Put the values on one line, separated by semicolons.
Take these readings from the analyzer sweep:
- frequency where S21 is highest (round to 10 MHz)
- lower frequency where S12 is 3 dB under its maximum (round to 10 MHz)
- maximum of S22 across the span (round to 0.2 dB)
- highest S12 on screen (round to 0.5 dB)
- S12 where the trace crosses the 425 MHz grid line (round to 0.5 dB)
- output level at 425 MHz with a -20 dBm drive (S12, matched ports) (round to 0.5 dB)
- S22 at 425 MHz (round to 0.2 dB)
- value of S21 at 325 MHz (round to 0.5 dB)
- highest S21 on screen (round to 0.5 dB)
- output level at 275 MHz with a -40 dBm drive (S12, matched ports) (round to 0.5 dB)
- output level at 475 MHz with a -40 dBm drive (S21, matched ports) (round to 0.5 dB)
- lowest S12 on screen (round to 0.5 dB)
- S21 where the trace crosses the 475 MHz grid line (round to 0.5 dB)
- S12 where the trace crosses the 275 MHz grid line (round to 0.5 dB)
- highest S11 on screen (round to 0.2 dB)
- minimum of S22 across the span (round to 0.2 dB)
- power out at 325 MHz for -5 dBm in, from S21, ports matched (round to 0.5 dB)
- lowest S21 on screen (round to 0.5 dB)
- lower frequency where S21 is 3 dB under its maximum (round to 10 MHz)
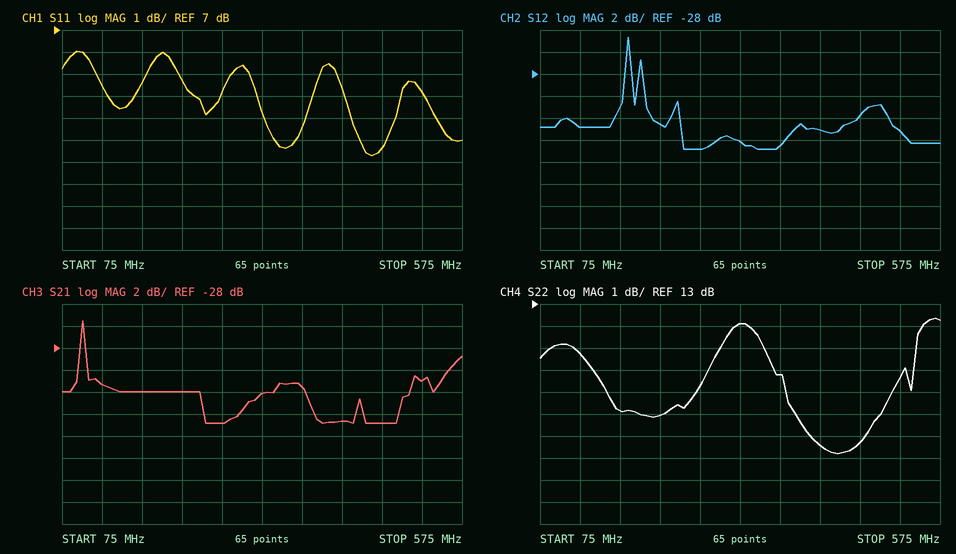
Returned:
100 MHz; 180 MHz; 12.4 dB; -24.5 dB; -33.0 dB; -53.0 dBm; 6.6 dB; -32.0 dB; -25.5 dB; -75.0 dBm; -75.0 dBm; -35.0 dB; -35.0 dB; -35.0 dB; 6.0 dB; 6.2 dB; -37.0 dBm; -35.0 dB; 100 MHz
